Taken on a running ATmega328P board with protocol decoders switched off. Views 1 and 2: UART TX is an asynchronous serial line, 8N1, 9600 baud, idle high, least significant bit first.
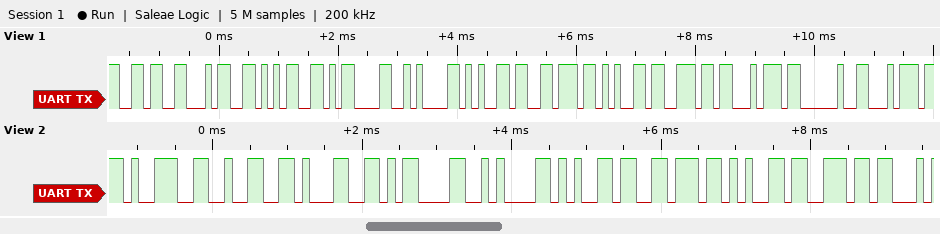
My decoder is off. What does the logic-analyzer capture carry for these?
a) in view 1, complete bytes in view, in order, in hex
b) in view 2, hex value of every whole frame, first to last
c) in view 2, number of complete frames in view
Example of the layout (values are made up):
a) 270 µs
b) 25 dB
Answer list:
a) 0x36 0x34 0x35 0x0D 0x0A 0x65 0x76 0x65 0x6E 0x74 0x20 0x74
b) 0x39 0x32 0x31 0x0D 0x0A 0x65 0x76 0x65 0x6E
c) 9
